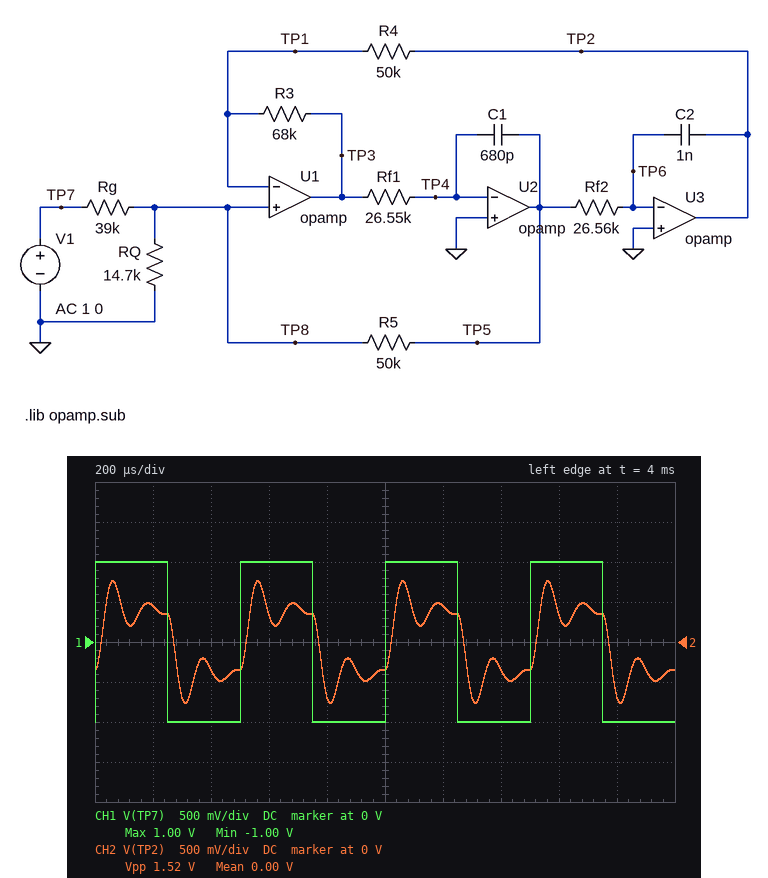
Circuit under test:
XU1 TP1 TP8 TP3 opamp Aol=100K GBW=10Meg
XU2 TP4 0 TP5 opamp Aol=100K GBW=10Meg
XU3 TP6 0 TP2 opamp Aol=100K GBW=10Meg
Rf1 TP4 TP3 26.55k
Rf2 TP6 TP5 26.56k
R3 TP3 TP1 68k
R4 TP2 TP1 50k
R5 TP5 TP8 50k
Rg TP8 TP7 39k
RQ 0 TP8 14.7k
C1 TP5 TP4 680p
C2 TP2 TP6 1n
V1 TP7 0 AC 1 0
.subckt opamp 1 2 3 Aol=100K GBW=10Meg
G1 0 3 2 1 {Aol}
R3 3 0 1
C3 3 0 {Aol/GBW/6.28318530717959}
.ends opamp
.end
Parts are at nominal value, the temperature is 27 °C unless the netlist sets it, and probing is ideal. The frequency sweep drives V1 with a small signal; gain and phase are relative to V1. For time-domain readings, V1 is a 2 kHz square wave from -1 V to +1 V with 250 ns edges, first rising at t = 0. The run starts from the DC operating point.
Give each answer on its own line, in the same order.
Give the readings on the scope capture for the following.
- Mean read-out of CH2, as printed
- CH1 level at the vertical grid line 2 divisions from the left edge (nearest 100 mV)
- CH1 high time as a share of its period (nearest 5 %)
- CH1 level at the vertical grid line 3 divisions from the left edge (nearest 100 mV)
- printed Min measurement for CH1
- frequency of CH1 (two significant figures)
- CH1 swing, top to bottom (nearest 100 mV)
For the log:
0.00 V
-1.0 V
50 %
1.0 V
-1.00 V
2.0 kHz
2.0 V
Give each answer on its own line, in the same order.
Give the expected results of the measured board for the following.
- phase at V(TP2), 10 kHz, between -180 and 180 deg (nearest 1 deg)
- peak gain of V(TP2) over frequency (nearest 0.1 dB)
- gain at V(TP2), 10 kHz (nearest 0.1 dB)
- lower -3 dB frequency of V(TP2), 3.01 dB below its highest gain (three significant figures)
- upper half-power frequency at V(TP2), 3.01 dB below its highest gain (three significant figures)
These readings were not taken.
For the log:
-128 deg
-0.6 dB
-4.3 dB
5.93 kHz
9.76 kHz
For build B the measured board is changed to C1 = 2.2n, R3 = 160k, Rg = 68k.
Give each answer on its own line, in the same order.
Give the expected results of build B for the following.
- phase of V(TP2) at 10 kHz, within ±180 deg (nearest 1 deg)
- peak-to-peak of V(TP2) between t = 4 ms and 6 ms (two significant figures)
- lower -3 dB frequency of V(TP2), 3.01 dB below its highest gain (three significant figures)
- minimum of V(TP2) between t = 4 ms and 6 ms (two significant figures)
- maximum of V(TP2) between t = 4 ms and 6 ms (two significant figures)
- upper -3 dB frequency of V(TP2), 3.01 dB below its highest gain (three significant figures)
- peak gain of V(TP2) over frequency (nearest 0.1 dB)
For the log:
-156 deg
830 mV
5.84 kHz
-410 mV
410 mV
8.10 kHz
-4.1 dB
